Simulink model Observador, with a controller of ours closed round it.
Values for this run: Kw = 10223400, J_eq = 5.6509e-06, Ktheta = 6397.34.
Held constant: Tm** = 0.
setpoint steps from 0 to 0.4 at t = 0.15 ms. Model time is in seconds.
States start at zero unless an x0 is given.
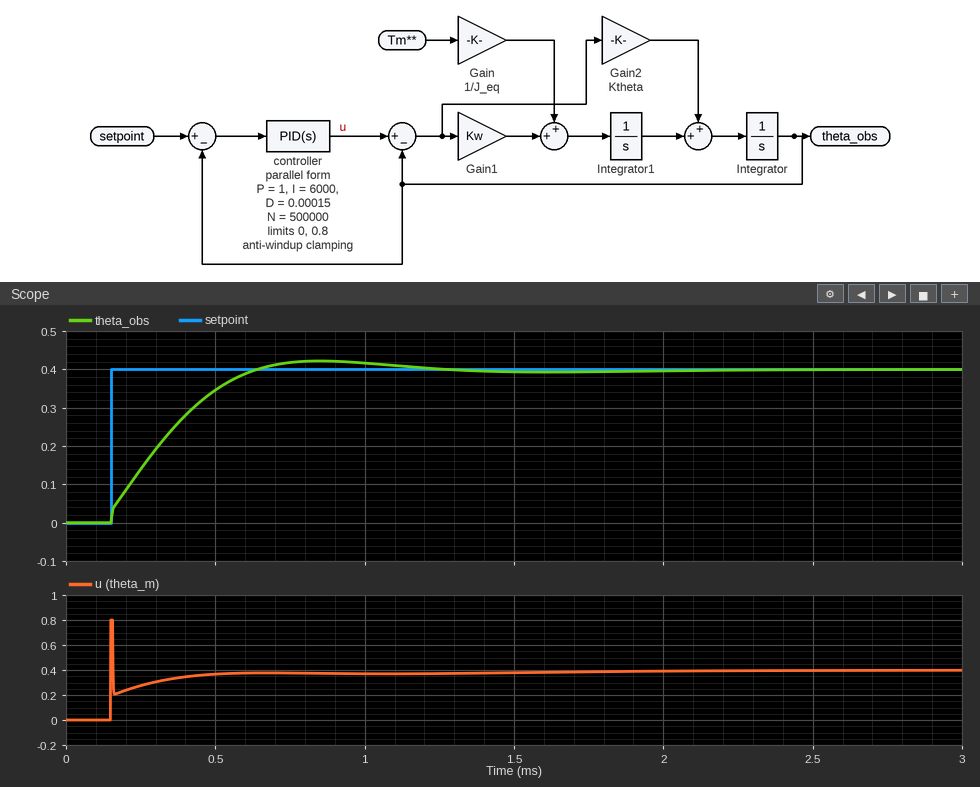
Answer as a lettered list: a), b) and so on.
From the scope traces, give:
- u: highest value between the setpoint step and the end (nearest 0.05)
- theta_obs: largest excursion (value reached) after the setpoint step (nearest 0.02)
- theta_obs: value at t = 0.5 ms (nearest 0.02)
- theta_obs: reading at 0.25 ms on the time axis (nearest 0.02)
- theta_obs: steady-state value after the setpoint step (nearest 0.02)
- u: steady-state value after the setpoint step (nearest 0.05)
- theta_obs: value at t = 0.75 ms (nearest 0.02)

a) 0.80
b) 0.42
c) 0.34
d) 0.14
e) 0.40
f) 0.40
g) 0.42
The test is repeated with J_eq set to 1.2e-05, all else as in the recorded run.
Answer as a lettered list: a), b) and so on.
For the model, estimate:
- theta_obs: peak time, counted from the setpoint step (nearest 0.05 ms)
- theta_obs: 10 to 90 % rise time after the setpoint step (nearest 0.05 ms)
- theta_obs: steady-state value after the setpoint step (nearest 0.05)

a) 0.70 ms
b) 0.35 ms
c) 0.40
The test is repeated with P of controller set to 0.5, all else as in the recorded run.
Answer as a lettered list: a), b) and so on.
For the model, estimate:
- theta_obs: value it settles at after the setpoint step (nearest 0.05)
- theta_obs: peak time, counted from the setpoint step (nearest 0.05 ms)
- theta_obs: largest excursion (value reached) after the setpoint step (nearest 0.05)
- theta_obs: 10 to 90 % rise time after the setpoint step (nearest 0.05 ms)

a) 0.40
b) 0.70 ms
c) 0.45
d) 0.40 ms
